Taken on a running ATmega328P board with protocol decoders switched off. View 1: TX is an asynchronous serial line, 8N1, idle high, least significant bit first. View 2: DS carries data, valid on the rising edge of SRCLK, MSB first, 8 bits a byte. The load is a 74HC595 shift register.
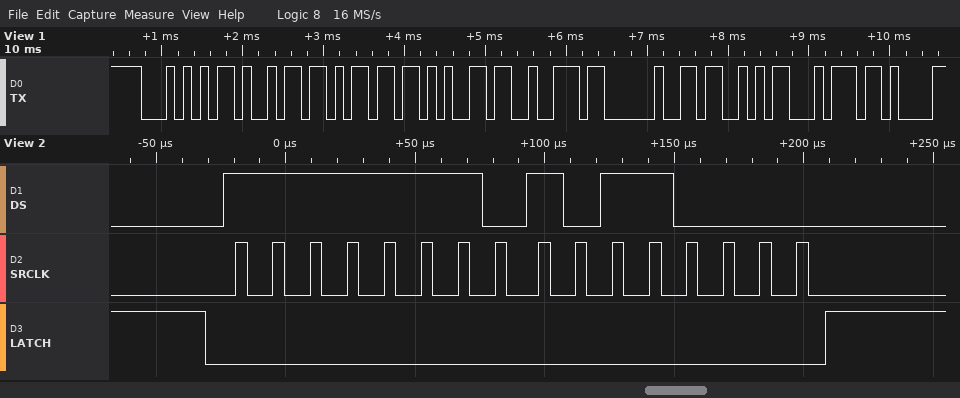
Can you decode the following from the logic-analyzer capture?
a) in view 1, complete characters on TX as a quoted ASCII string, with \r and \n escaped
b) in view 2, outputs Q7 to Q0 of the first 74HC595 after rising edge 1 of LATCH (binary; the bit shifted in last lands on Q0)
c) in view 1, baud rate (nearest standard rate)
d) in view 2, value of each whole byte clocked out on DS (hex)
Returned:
"Timer St"
10110000
9600 baud
FE B0
